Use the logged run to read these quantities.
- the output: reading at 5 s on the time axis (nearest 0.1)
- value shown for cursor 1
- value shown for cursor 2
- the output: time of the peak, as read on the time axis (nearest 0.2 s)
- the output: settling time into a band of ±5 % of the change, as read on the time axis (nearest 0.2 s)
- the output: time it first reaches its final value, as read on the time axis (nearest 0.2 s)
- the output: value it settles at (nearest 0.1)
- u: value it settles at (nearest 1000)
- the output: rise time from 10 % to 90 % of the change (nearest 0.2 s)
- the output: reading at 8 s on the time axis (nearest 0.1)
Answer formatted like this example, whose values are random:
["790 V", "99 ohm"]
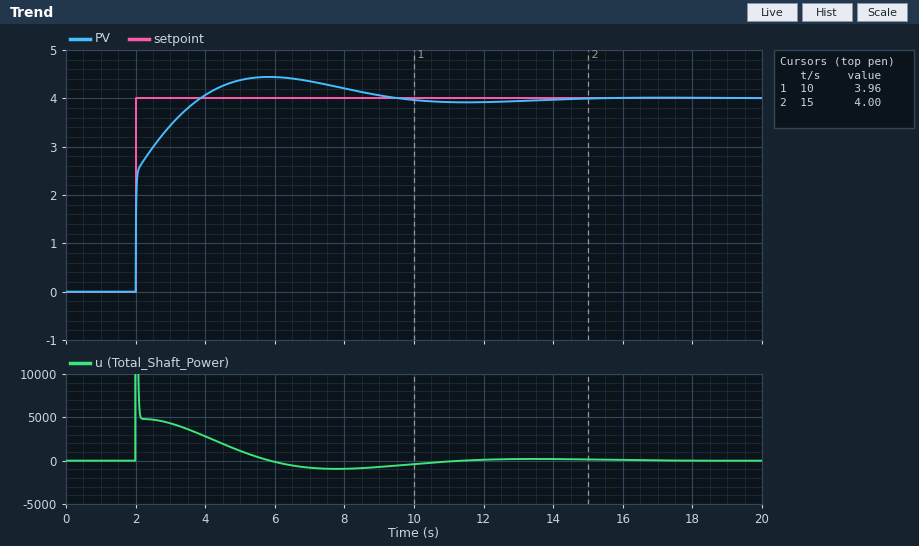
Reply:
["4.4", "3.96", "4.00", "5.8 s", "8.0 s", "3.8 s", "4.0", "0", "1.2 s", "4.2"]
